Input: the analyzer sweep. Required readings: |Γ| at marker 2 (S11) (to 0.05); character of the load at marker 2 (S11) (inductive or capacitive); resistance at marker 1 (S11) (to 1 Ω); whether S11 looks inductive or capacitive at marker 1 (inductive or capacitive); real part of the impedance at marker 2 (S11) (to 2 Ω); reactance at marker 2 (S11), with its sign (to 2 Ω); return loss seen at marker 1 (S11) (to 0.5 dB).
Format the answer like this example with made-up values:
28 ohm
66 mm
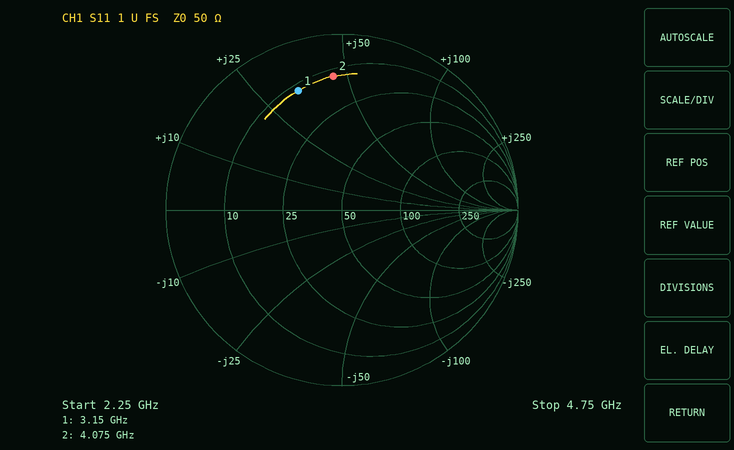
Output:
0.75
inductive
12 Ω
inductive
12 Ω
+46 Ω
3.0 dB
